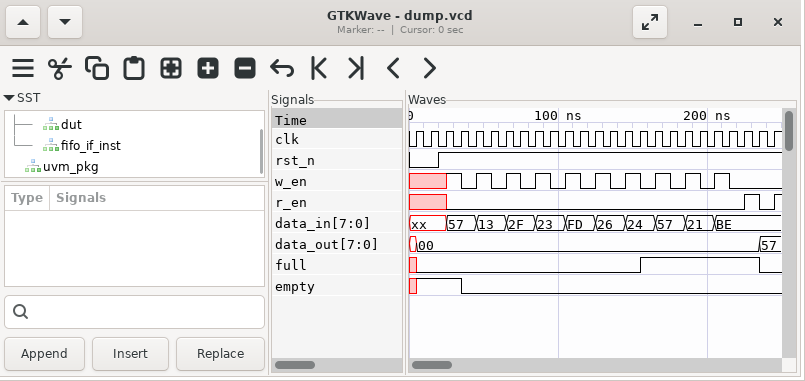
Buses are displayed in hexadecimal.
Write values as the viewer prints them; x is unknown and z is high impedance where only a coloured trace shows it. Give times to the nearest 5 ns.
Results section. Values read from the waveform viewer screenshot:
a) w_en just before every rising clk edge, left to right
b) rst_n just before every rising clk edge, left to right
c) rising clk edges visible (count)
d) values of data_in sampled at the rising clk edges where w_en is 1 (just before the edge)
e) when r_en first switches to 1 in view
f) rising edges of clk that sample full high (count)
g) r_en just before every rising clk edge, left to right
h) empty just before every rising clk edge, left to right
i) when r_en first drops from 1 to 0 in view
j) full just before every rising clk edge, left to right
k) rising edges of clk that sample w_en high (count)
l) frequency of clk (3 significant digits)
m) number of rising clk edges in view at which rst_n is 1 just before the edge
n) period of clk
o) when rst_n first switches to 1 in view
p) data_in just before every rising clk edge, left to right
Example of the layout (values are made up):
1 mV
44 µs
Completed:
x x x 1 0 1 0 1 0 1 0 1 0 1 0 1 0 1 0 1 0 1 0 0 0
0 0 1 1 1 1 1 1 1 1 1 1 1 1 1 1 1 1 1 1 1 1 1 1 1
25
57, 13, 2F, 23, FD, 26, 24, 57, 21, BE
225 ns
8
x x x 0 0 0 0 0 0 0 0 0 0 0 0 0 0 0 0 0 0 0 0 1 0
x 1 1 1 0 0 0 0 0 0 0 0 0 0 0 0 0 0 0 0 0 0 0 0 0
235 ns
x 0 0 0 0 0 0 0 0 0 0 0 0 0 0 0 1 1 1 1 1 1 1 1 0
10
100 MHz
23
10 ns
20 ns
xx, xx, xx, 57, 57, 13, 13, 2F, 2F, 23, 23, FD, FD, 26, 26, 24, 24, 57, 57, 21, 21, BE, BE, BE, BE
